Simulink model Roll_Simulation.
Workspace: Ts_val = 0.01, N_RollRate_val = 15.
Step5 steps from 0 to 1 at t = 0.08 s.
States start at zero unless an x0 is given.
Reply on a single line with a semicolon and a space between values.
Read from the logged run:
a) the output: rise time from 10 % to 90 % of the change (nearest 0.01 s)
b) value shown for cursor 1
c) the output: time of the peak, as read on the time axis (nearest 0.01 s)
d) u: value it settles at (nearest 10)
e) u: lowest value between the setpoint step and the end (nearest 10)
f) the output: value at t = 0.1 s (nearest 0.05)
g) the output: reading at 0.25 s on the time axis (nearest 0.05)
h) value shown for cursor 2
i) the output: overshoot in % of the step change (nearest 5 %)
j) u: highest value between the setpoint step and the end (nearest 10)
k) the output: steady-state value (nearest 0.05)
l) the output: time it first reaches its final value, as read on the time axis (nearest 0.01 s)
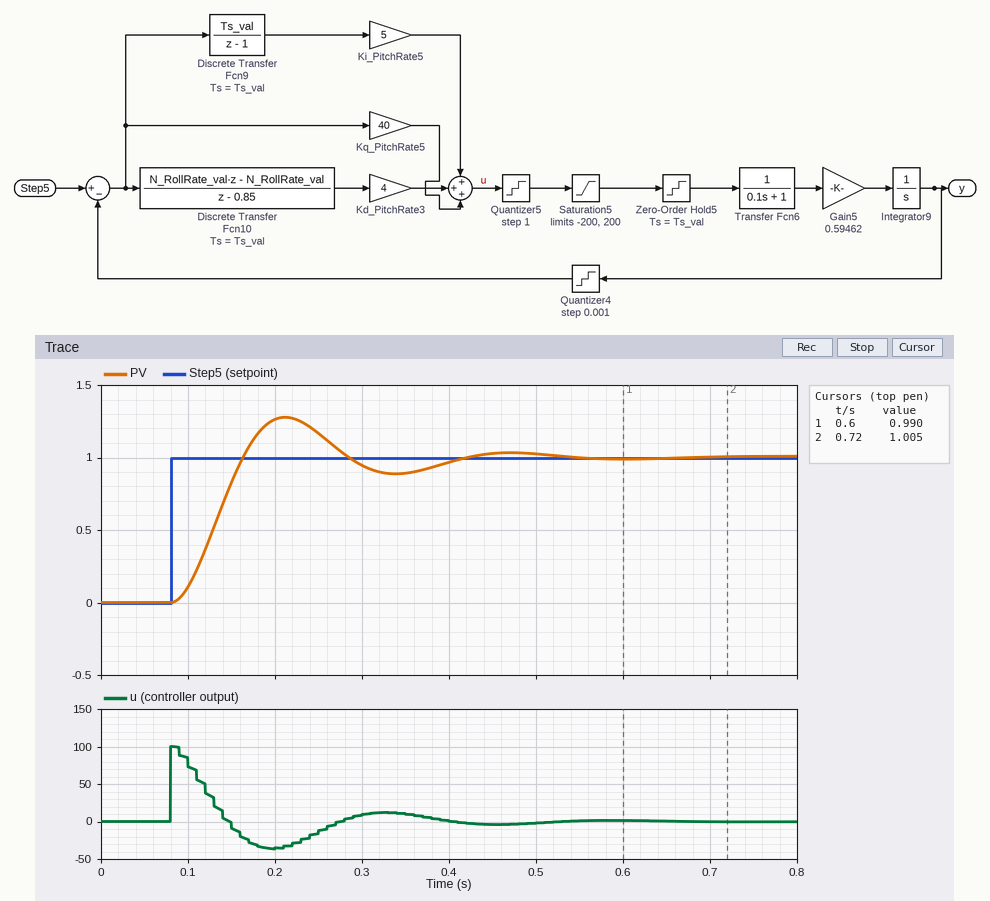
0.06 s; 0.990; 0.21 s; 0; -40; 0.10; 1.15; 1.005; 25 %; 100; 1.00; 0.16 s
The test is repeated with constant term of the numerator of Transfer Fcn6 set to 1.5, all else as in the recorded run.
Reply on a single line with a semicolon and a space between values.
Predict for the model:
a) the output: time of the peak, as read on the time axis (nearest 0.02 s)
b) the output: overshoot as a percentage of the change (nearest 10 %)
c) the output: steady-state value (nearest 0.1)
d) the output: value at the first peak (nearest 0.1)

0.18 s; 40 %; 1.0; 1.4
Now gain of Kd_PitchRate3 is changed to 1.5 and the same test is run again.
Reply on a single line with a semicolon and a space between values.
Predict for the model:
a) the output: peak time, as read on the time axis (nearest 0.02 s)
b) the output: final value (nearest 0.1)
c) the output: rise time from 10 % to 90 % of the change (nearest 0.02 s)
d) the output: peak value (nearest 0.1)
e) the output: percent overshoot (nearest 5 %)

0.26 s; 1.0; 0.08 s; 1.3; 30 %
